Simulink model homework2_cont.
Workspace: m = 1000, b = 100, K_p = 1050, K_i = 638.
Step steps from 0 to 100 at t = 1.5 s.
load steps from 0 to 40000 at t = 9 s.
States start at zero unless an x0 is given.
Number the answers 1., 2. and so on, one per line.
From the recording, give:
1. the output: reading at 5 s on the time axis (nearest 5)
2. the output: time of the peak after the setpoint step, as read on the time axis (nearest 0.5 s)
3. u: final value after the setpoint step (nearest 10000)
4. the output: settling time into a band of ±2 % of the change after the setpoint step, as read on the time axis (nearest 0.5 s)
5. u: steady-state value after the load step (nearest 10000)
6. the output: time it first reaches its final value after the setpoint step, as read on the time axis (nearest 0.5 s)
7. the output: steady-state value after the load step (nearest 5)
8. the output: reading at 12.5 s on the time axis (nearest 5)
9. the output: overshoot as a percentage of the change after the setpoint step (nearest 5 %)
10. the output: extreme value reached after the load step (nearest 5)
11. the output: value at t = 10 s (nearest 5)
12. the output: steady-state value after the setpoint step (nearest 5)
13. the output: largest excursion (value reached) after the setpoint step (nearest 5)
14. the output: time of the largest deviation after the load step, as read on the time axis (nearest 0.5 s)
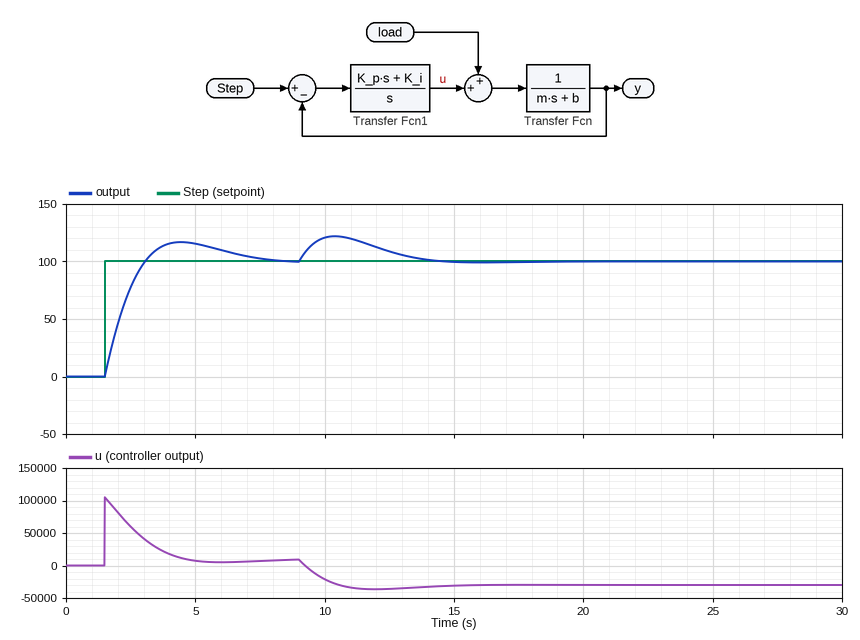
1. 115
2. 4.5 s
3. 10000
4. 7.5 s
5. -30000
6. 3.0 s
7. 100
8. 110
9. 15 %
10. 120
11. 120
12. 100
13. 115
14. 10.5 s
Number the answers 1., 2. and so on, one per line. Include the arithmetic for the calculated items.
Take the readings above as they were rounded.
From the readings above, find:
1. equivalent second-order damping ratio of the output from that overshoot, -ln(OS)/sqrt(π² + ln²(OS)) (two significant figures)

1. ln(0.15) = -1.897; 1.897 / sqrt(9.870 + 3.599) = 0.52
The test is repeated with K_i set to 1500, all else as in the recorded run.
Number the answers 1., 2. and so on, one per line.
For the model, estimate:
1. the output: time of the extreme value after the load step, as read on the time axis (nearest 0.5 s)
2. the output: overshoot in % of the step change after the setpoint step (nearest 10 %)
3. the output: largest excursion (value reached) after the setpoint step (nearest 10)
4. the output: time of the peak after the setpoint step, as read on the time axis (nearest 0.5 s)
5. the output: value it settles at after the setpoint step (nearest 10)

1. 10.0 s
2. 30 %
3. 130
4. 3.5 s
5. 100
